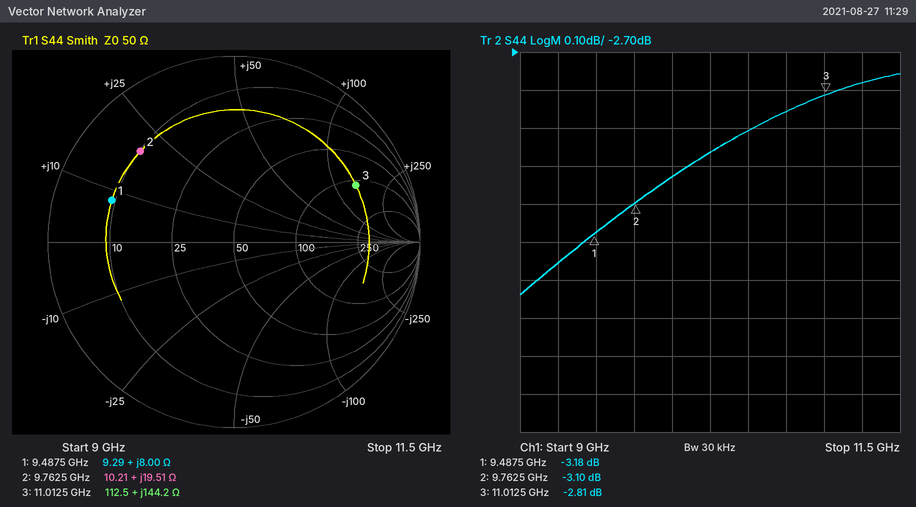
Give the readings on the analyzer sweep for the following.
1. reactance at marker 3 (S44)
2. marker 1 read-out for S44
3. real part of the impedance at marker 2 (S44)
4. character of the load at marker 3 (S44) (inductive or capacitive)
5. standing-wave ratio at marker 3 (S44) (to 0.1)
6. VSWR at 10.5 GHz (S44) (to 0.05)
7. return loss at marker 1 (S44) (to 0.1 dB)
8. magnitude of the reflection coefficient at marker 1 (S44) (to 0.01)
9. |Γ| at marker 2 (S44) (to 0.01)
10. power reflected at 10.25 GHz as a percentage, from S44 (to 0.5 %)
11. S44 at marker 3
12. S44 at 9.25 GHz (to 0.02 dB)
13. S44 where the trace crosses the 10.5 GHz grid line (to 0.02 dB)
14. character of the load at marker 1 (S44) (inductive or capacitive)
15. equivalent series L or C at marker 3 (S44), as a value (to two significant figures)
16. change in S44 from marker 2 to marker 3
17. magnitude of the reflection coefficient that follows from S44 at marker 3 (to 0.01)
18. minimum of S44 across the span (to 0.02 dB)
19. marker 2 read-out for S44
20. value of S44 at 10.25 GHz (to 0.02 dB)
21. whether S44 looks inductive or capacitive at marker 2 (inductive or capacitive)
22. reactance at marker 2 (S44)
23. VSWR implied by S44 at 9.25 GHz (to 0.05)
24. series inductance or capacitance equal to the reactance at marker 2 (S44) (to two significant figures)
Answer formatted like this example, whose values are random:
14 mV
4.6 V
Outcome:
+144.2 Ω
-3.18 dB
10.21 Ω
inductive
6.2
6.05
3.2 dB
0.69
0.70
50.5 %
-2.81 dB
-3.26 dB
-2.90 dB
inductive
2.1 nH
0.29 dB
0.72
-3.34 dB
-3.10 dB
-2.96 dB
inductive
+19.51 Ω
5.40
320 pH
